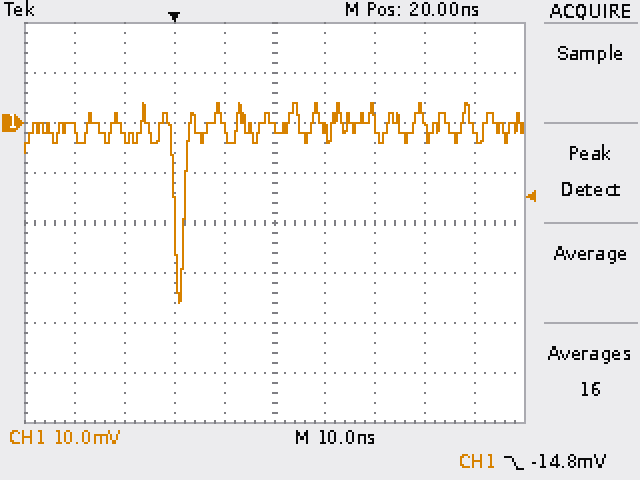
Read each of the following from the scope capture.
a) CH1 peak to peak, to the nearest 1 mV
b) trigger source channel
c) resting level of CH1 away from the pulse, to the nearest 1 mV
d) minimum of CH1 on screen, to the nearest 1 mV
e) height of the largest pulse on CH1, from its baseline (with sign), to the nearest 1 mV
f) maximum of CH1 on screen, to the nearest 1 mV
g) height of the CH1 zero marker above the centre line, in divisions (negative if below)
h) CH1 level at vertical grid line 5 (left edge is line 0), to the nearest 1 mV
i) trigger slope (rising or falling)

40 mV
CH1
-1 mV
-36 mV
-35 mV
4 mV
+2.0 div
-1 mV
falling
